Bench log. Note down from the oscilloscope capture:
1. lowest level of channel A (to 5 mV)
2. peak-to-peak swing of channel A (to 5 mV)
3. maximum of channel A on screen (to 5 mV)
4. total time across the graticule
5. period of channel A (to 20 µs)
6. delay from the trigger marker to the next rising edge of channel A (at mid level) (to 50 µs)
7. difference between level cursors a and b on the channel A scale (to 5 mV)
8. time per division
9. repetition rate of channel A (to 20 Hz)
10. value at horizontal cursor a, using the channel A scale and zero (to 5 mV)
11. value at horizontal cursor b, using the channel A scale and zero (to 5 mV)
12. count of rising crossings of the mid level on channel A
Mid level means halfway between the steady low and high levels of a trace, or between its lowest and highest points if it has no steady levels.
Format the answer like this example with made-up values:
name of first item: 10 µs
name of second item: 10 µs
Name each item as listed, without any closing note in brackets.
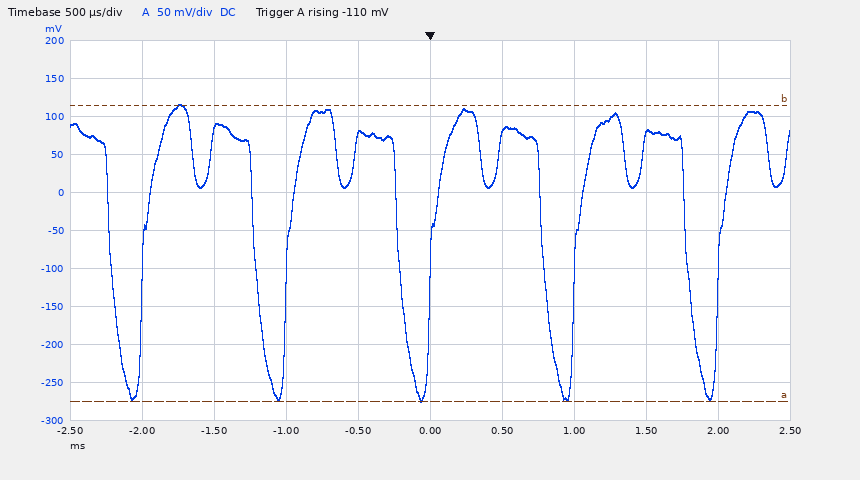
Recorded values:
lowest level of channel A: -275 mV
peak-to-peak swing of channel A: 390 mV
maximum of channel A on screen: 115 mV
total time across the graticule: 5 ms
period of channel A: 1.00 ms
delay from the trigger marker to the next rising edge of channel A (at mid level): 1.00 ms
difference between level cursors a and b on the channel A scale: 390 mV
time per division: 500 µs
repetition rate of channel A: 1.00 kHz
value at horizontal cursor a, using the channel A scale and zero: -275 mV
value at horizontal cursor b, using the channel A scale and zero: 115 mV
count of rising crossings of the mid level on channel A: 5
